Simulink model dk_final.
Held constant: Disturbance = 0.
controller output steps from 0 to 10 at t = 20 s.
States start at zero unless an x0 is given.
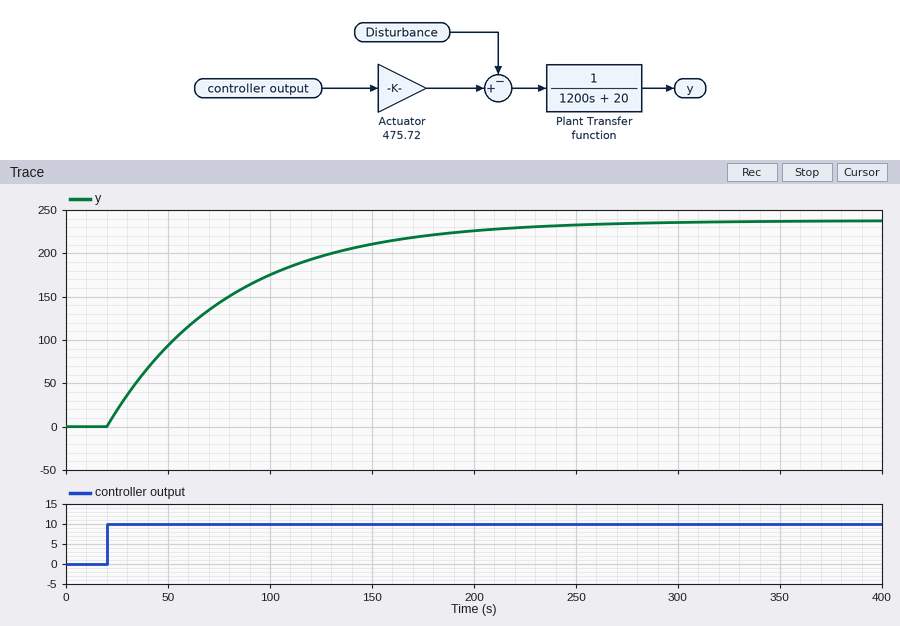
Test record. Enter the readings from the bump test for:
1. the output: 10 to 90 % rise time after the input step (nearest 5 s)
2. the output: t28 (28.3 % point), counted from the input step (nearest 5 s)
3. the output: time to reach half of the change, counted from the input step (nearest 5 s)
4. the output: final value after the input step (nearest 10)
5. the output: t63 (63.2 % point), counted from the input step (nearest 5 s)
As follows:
130 s
20 s
40 s
240
60 s
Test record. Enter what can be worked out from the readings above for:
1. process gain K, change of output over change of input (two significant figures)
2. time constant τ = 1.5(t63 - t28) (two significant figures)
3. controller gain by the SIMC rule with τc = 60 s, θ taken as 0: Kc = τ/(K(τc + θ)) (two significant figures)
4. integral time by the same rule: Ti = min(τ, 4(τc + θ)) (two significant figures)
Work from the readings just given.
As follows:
24
60 s
0.042
60 s
